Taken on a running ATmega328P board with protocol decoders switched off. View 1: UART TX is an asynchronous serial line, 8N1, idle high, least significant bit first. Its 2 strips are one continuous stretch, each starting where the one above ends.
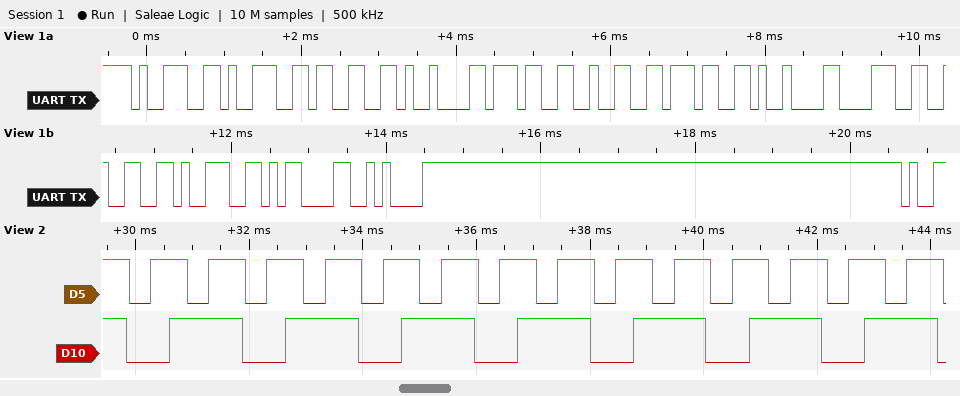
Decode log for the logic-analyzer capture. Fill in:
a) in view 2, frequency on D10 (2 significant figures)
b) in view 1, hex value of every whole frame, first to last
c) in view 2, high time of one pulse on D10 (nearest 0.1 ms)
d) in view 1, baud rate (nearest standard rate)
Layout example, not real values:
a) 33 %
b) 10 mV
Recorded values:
a) 490 Hz
b) 0x39 0x39 0x33 0x09 0x37 0x32 0x37 0x09 0x38 0x32 0x39 0x0D 0x0A
c) 1.3 ms
d) 9600 baud
